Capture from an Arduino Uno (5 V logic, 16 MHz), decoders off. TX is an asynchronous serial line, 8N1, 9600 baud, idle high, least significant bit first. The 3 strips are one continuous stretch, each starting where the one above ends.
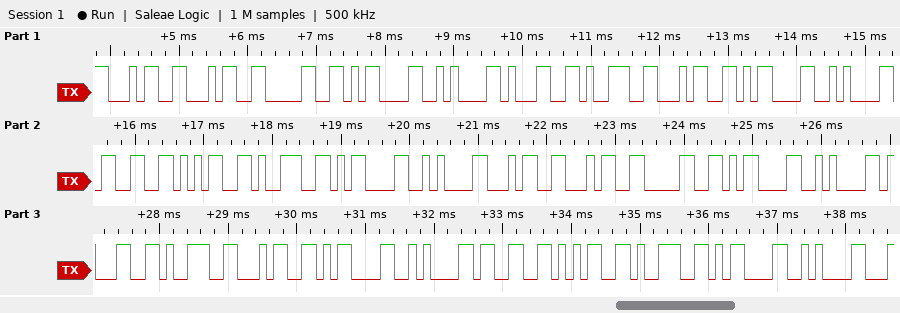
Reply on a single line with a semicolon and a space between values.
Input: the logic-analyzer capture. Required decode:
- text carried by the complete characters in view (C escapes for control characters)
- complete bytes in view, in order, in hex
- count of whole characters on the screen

"440\r\n194\r\n359\r\n440\r\n194\r\n359\r\n"; 34 34 30 0D 0A 31 39 34 0D 0A 33 35 39 0D 0A 34 34 30 0D 0A 31 39 34 0D 0A 33 35 39 0D 0A; 30
